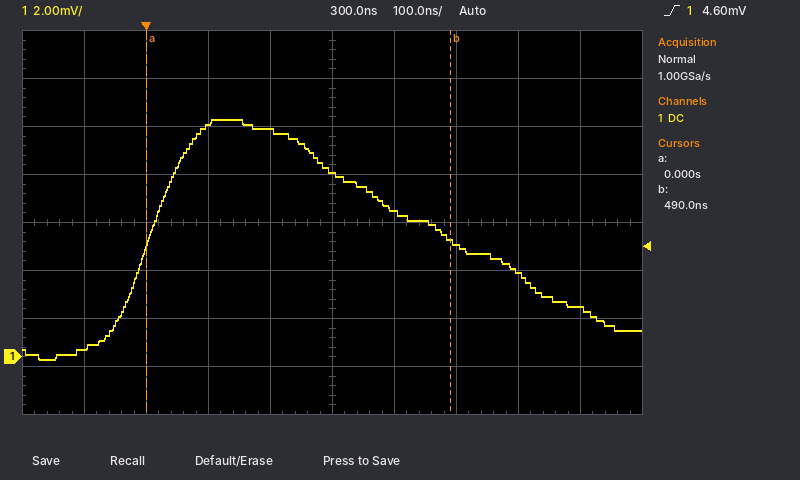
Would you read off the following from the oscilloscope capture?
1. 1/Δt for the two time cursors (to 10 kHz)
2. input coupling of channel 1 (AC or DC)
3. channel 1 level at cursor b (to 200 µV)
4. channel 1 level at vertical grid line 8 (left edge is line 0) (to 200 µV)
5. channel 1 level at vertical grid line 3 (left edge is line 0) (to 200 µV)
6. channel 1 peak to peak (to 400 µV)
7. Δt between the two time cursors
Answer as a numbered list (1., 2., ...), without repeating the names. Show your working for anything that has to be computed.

1. 1 / 490 ns ≈ 2.04 MHz
2. DC
3. 4.8 mV
4. 3.6 mV
5. 9.6 mV
6. 10.0 mV
7. 490 ns − (0 s) = 490 ns
